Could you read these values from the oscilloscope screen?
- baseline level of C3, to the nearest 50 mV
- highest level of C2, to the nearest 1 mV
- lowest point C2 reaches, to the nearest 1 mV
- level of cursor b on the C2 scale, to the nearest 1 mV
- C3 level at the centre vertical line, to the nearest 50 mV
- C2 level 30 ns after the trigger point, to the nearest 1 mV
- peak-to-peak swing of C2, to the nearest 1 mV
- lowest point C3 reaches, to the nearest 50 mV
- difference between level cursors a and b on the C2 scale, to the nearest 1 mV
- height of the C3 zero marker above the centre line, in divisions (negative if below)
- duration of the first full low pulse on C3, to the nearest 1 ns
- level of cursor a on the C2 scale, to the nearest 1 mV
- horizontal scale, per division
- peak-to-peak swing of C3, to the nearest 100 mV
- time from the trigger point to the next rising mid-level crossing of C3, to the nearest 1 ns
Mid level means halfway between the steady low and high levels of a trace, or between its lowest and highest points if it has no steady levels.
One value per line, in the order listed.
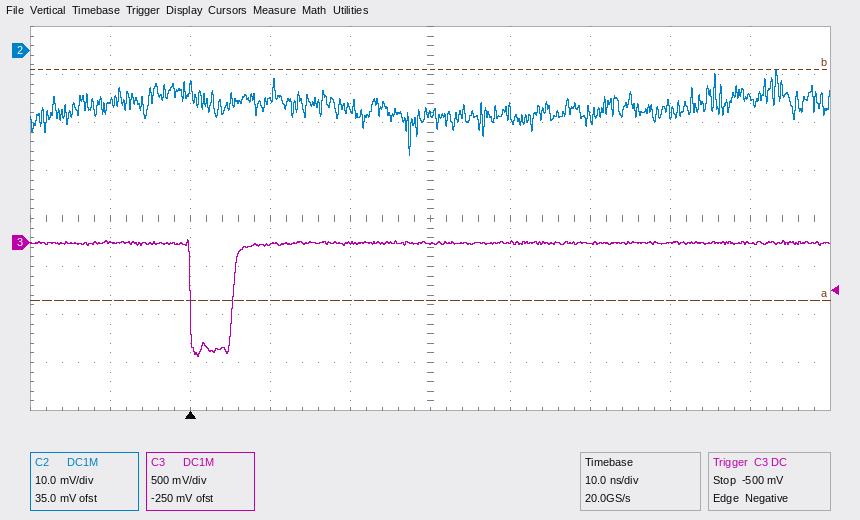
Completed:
0 mV
-4 mV
-22 mV
-4 mV
0 mV
-13 mV
18 mV
-1.20 V
48 mV
-0.5 div
5 ns
-52 mV
10 ns
1.20 V
5 ns
